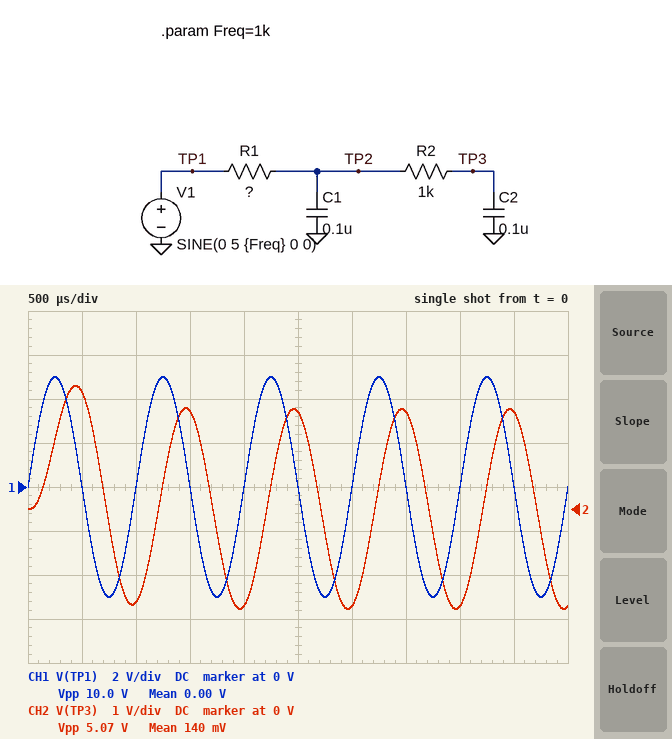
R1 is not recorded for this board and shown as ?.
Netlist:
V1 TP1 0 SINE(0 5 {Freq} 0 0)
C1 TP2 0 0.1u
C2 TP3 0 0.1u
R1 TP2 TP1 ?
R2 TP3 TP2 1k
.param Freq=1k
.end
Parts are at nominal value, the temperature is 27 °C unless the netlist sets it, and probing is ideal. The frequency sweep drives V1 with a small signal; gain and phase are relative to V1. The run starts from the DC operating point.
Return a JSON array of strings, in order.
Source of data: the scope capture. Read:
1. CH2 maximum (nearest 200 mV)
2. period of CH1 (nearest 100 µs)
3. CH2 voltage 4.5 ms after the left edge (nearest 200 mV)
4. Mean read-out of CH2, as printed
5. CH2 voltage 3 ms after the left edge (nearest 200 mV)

["2.8 V", "1.0 ms", "2.2 V", "140 mV", "-2.2 V"]
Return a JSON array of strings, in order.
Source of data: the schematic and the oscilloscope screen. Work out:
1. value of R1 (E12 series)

["1.2 kΩ"]
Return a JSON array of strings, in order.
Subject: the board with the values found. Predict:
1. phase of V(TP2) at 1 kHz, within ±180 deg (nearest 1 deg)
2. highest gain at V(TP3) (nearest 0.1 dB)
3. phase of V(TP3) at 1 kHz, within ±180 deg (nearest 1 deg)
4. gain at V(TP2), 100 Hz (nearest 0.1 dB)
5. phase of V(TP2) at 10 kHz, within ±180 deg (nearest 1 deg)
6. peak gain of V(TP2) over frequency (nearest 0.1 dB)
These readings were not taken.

["-44 deg", "0 dB", "-76 deg", "-0.1 dB", "-74 deg", "0 dB"]
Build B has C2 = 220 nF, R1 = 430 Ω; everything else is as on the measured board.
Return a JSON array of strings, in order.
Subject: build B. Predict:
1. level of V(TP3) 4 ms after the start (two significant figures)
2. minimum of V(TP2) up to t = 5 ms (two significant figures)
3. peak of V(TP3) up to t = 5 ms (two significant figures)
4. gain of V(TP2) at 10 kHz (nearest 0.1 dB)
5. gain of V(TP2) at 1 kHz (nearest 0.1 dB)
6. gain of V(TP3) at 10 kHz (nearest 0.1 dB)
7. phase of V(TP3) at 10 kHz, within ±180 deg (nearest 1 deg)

["-2.1 V", "-3.7 V", "2.7 V", "-9.8 dB", "-2.7 dB", "-32.6 dB", "-148 deg"]
